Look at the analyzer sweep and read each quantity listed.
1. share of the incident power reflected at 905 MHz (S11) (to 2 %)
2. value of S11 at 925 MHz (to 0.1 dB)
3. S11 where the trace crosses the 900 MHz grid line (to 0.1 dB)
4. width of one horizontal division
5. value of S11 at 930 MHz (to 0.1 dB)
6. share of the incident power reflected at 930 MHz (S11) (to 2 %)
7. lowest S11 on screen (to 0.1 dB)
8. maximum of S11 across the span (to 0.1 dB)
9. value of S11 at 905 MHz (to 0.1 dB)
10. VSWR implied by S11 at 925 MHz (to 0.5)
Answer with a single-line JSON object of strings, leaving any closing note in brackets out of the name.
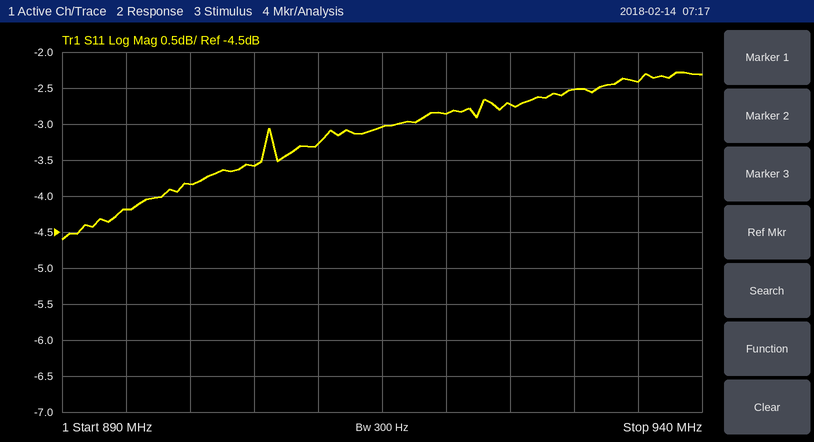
{"share of the incident power reflected at 905 MHz (S11)": "44 %", "value of S11 at 925 MHz": "-2.7 dB", "S11 where the trace crosses the 900 MHz grid line": "-3.8 dB", "width of one horizontal division": "5 MHz", "value of S11 at 930 MHz": "-2.5 dB", "share of the incident power reflected at 930 MHz (S11)": "56 %", "lowest S11 on screen": "-4.6 dB", "maximum of S11 across the span": "-2.3 dB", "value of S11 at 905 MHz": "-3.6 dB", "VSWR implied by S11 at 925 MHz": "6.5"}
